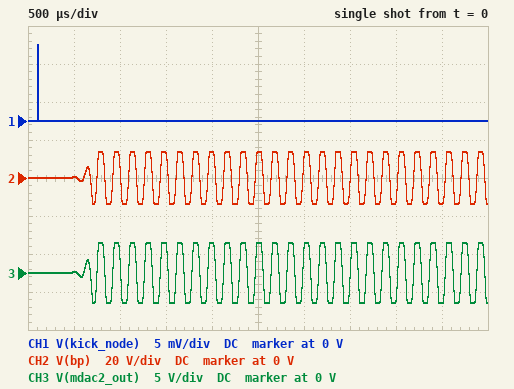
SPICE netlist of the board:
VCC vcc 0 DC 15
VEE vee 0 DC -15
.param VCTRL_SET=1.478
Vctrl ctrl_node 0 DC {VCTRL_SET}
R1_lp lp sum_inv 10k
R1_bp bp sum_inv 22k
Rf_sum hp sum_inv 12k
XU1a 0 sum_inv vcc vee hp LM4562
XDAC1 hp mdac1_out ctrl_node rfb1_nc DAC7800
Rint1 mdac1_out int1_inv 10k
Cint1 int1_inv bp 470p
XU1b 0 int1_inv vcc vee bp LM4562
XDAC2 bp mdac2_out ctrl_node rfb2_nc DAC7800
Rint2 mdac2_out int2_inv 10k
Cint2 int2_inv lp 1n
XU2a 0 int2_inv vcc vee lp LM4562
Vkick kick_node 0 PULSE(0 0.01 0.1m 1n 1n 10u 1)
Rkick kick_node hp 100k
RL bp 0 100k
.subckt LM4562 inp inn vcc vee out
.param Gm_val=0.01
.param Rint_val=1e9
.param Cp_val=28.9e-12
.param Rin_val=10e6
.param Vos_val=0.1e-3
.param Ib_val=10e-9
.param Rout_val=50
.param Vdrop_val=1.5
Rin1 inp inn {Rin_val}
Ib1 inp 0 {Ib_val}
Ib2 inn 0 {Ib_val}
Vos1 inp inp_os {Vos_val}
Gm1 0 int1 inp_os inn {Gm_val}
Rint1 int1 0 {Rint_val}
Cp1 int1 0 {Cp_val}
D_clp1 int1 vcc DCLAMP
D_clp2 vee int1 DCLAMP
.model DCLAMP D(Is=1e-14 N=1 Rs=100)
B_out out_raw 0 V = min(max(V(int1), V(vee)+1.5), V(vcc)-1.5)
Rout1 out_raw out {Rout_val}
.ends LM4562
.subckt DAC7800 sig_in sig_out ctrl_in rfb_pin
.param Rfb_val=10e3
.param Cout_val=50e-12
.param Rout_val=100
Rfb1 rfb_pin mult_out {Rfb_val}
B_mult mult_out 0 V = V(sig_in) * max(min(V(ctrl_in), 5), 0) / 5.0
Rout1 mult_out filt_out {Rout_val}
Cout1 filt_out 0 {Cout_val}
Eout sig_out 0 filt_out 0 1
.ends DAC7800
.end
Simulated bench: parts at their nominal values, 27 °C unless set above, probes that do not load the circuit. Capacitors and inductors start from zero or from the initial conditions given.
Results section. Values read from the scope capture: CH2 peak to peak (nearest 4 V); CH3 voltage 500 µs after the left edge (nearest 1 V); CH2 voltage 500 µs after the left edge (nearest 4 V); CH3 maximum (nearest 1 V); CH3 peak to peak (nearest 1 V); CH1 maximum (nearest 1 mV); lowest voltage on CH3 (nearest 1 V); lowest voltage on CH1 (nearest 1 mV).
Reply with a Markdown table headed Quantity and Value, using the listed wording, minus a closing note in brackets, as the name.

| Quantity | Value |
|---|---|
| CH2 peak to peak | 28 V |
| CH3 voltage 500 µs after the left edge | 0 V |
| CH2 voltage 500 µs after the left edge | 0 V |
| CH3 maximum | 4 V |
| CH3 peak to peak | 8 V |
| CH1 maximum | 10 mV |
| lowest voltage on CH3 | -4 V |
| lowest voltage on CH1 | 0 V |
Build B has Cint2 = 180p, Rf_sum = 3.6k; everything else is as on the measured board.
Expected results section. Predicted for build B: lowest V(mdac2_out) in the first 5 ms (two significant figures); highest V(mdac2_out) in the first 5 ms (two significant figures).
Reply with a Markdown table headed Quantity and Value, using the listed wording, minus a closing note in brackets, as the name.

| Quantity | Value |
|---|---|
| lowest V(mdac2_out) in the first 5 ms | -1.7 V |
| highest V(mdac2_out) in the first 5 ms | 1.7 V |
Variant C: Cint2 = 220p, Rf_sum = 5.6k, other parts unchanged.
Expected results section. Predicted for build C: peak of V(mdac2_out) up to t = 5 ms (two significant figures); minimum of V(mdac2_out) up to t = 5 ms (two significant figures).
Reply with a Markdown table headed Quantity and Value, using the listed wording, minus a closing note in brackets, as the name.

| Quantity | Value |
|---|---|
| peak of V(mdac2_out) up to t = 5 ms | 2.5 V |
| minimum of V(mdac2_out) up to t = 5 ms | -2.5 V |
